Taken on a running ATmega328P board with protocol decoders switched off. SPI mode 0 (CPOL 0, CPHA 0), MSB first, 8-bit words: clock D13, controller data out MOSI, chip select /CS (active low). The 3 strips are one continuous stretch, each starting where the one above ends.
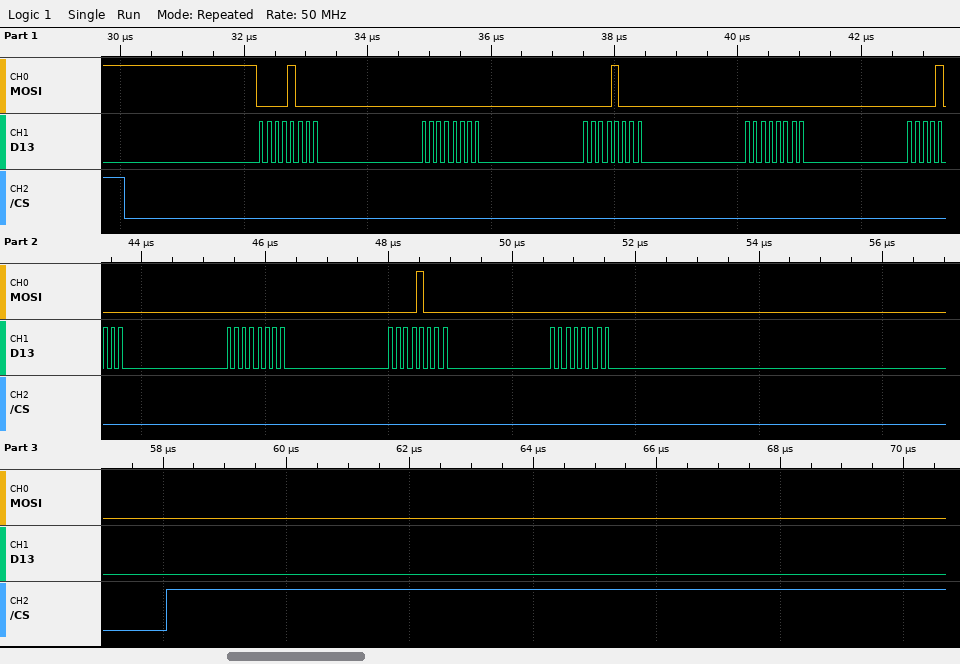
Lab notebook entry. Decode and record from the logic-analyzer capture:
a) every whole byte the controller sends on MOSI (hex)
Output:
0x08 0x00 0x08 0x00 0x08 0x00 0x08 0x00
